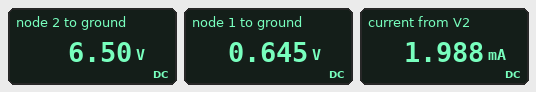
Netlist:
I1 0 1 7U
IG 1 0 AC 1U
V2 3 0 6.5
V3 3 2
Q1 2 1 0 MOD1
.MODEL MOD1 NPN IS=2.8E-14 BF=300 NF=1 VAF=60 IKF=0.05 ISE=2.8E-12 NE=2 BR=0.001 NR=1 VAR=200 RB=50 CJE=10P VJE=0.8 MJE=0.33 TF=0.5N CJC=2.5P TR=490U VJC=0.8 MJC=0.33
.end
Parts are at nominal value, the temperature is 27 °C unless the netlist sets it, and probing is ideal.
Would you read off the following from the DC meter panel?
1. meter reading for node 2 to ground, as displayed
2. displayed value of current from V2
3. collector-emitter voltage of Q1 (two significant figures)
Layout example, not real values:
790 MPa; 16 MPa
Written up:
6.50 V; 1.988 mA; 6.5 V
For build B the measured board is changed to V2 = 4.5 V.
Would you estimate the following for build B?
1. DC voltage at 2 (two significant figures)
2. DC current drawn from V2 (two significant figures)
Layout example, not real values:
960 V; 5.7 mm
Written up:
4.5 V; 1.9 mA
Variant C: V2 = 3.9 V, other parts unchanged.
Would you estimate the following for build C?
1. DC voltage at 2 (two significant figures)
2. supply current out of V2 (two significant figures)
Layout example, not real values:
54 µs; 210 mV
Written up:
3.9 V; 1.9 mA
